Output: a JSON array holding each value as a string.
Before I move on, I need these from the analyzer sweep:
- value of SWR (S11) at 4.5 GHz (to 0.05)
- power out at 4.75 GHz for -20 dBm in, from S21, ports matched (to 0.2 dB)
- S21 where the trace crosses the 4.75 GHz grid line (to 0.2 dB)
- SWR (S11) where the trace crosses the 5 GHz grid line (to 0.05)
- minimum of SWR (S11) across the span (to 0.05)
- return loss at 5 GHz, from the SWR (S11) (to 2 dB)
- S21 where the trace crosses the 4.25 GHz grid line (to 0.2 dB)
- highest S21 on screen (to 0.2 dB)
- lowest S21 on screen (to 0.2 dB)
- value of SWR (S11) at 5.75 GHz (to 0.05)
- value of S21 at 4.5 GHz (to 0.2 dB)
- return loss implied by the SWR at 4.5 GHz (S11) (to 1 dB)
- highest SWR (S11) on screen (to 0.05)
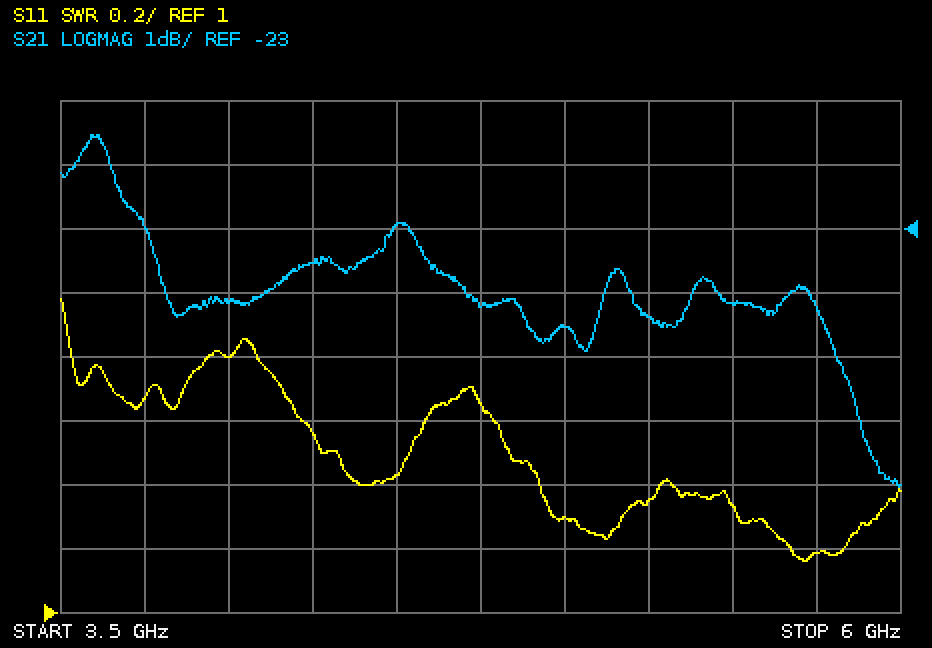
["1.45", "-44.2 dBm", "-24.2 dB", "1.30", "1.15", "18 dB", "-23.6 dB", "-21.6 dB", "-27.0 dB", "1.20", "-23.0 dB", "15 dB", "2.00"]
